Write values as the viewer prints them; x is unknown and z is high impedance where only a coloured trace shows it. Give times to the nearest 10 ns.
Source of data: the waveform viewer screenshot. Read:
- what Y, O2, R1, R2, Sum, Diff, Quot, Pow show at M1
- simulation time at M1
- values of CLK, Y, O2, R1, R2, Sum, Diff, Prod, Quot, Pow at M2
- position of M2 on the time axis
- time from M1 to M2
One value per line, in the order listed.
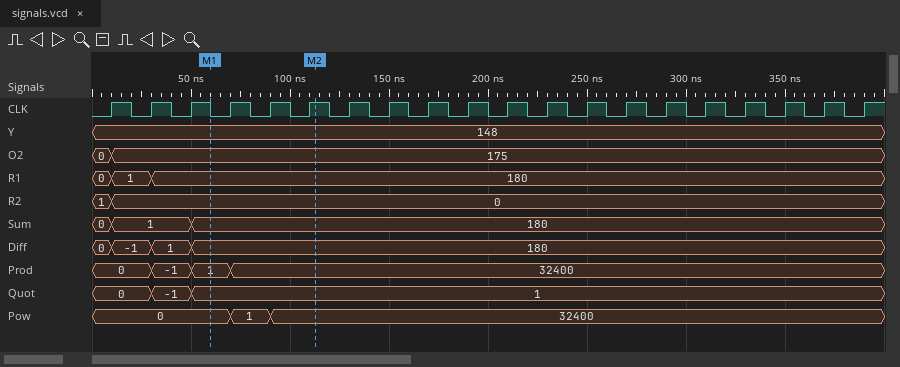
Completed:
Y=148, O2=175, R1=180, R2=0, Sum=180, Diff=180, Quot=1, Pow=0
60 ns
CLK=1, Y=148, O2=175, R1=180, R2=0, Sum=180, Diff=180, Prod=32400, Quot=1, Pow=32400
110 ns
50 ns
